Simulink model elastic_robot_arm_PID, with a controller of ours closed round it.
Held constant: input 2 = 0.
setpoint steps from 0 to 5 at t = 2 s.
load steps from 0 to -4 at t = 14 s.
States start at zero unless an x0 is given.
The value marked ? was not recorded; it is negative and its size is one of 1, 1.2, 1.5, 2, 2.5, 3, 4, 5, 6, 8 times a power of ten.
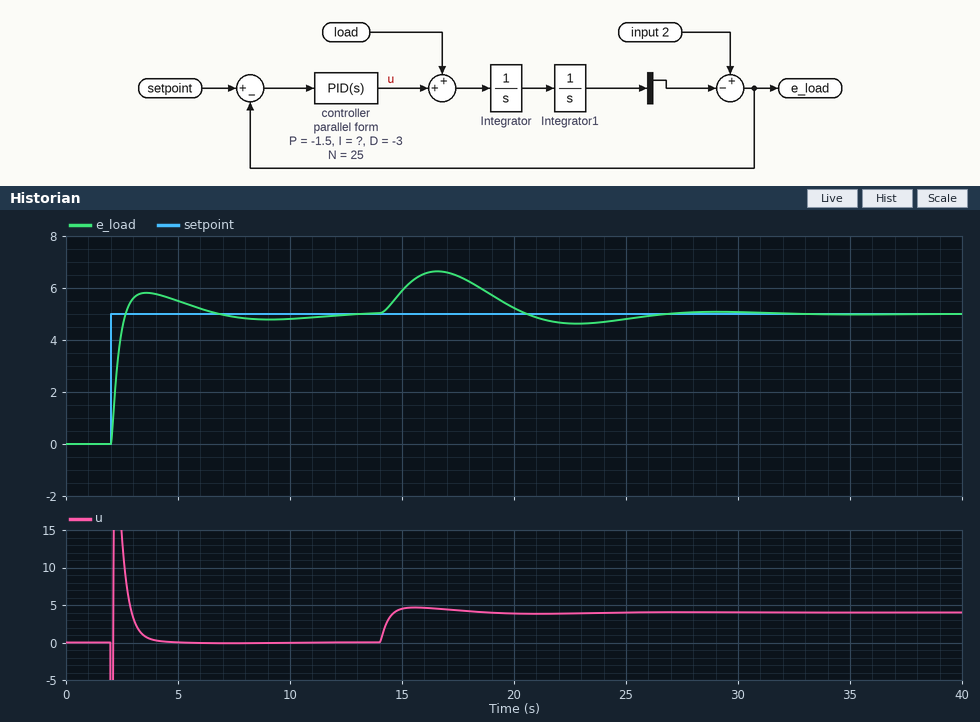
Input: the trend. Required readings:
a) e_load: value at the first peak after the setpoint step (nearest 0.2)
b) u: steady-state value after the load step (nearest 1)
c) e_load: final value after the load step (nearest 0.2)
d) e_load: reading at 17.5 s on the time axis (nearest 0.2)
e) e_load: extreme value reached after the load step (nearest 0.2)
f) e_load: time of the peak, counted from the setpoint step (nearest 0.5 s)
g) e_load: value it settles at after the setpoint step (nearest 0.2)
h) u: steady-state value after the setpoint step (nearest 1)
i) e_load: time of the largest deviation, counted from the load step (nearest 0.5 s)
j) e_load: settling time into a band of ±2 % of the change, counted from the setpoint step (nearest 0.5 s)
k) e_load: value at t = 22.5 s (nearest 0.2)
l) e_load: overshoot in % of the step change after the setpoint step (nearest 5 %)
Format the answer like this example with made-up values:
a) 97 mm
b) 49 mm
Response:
a) 5.8
b) 4
c) 5.0
d) 6.4
e) 6.6
f) 1.5 s
g) 5.0
h) 0
i) 2.5 s
j) 9.5 s
k) 4.6
l) 15 %
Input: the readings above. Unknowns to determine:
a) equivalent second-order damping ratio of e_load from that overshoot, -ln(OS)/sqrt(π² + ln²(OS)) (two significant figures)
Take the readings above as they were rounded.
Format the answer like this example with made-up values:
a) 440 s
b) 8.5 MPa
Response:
a) 0.52
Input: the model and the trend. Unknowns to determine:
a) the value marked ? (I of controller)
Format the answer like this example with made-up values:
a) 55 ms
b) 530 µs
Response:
a) -0.8
